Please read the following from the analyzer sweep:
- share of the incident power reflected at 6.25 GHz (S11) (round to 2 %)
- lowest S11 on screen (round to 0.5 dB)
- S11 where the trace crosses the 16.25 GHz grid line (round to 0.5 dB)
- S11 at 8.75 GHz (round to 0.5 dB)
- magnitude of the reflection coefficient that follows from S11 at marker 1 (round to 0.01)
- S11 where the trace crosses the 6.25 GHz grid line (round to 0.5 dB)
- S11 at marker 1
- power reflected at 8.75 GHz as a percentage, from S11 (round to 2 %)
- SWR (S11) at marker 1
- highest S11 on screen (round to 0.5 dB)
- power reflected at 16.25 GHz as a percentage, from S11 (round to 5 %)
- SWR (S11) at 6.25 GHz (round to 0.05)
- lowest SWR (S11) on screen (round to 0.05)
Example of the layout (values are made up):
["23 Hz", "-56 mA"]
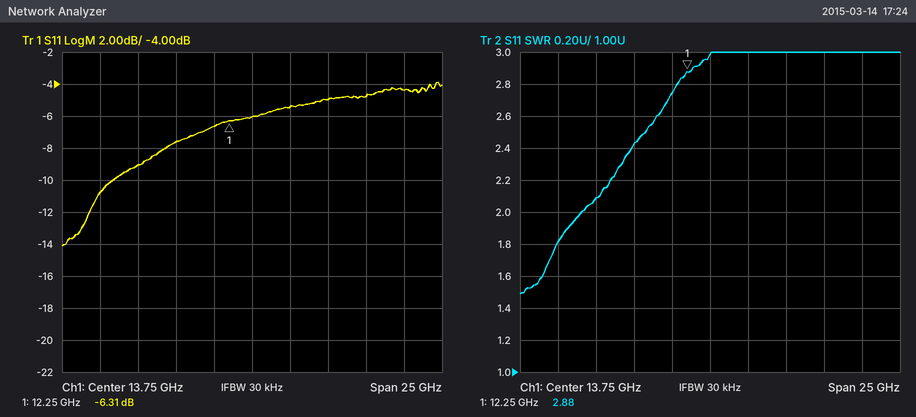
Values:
["12 %", "-14.0 dB", "-5.5 dB", "-7.5 dB", "0.48", "-9.0 dB", "-6.31 dB", "18 %", "2.88", "-4.0 dB", "30 %", "2.10", "1.50"]
